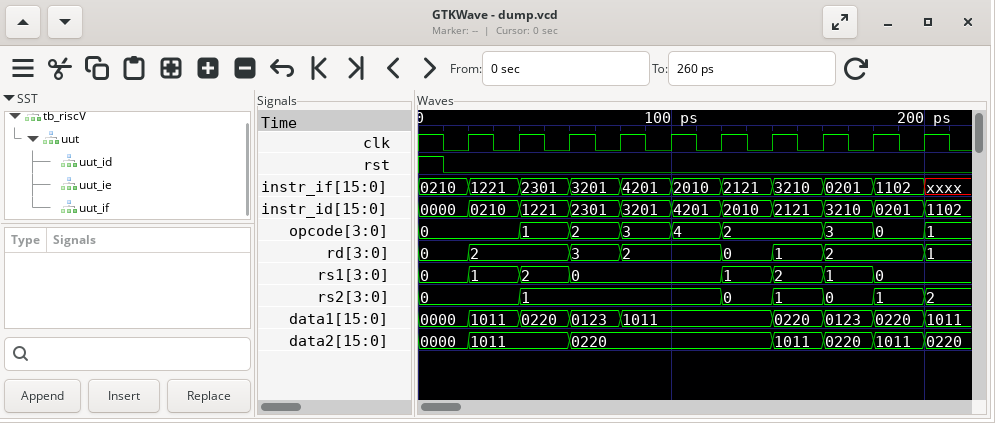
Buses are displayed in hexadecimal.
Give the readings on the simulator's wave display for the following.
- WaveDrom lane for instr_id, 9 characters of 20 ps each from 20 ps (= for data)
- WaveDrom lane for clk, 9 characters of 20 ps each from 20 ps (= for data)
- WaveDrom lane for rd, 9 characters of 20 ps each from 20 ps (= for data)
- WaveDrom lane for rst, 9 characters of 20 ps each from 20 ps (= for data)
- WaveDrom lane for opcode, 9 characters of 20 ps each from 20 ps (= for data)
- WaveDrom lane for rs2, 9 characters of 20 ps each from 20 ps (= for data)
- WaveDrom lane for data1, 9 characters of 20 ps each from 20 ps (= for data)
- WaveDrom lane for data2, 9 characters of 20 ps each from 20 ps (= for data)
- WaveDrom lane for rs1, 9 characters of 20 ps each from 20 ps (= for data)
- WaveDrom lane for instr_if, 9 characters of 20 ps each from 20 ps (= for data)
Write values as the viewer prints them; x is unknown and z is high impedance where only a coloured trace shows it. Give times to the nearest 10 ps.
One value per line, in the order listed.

{name: 'instr_id', wave: '=========', data: '0210 1221 2301 3201 4201 2010 2121 3210 0201'}
{name: 'clk', wave: 'p........'}
{name: 'rd', wave: '=.==.===.', data: '2 3 2 0 1 2'}
{name: 'rst', wave: '0........'}
{name: 'opcode', wave: '======.==', data: '0 1 2 3 4 2 3 0'}
{name: 'rs2', wave: '==...====', data: '0 1 0 1 0 1'}
{name: 'data1', wave: '====..===', data: '1011 0220 0123 1011 0220 0123 0220'}
{name: 'data2', wave: '=.=...===', data: '1011 0220 1011 0220 1011'}
{name: 'rs1', wave: '===..====', data: '1 2 0 1 2 1 0'}
{name: 'instr_if', wave: '=========', data: '1221 2301 3201 4201 2010 2121 3210 0201 1102'}
